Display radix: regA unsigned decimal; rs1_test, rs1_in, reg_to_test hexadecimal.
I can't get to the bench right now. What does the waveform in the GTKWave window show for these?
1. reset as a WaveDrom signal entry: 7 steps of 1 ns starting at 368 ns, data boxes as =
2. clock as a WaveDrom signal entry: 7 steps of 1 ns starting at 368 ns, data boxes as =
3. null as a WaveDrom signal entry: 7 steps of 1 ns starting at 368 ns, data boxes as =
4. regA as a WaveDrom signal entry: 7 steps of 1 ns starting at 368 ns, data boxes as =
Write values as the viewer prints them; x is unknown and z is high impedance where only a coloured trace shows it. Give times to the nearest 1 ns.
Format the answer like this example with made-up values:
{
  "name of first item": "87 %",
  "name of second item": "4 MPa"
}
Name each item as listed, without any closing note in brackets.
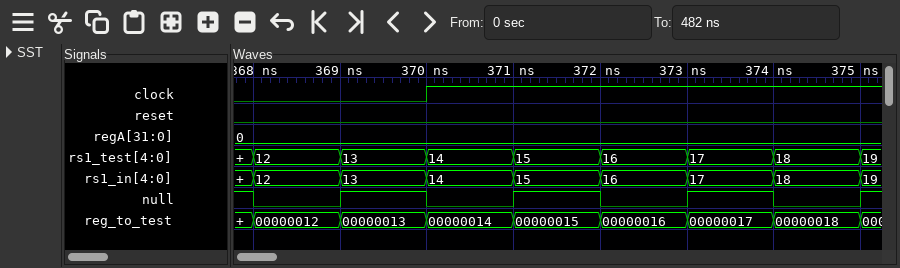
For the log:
{
  "reset as a WaveDrom signal entry: 7 steps of 1 ns starting at 368 ns, data boxes as =": "{name: 'reset', wave: '0......'}",
  "clock as a WaveDrom signal entry: 7 steps of 1 ns starting at 368 ns, data boxes as =": "{name: 'clock', wave: '0.1....'}",
  "null as a WaveDrom signal entry: 7 steps of 1 ns starting at 368 ns, data boxes as =": "{name: 'null', wave: '0101010'}",
  "regA as a WaveDrom signal entry: 7 steps of 1 ns starting at 368 ns, data boxes as =": "{name: 'regA', wave: '=......', data: '0'}"
}
